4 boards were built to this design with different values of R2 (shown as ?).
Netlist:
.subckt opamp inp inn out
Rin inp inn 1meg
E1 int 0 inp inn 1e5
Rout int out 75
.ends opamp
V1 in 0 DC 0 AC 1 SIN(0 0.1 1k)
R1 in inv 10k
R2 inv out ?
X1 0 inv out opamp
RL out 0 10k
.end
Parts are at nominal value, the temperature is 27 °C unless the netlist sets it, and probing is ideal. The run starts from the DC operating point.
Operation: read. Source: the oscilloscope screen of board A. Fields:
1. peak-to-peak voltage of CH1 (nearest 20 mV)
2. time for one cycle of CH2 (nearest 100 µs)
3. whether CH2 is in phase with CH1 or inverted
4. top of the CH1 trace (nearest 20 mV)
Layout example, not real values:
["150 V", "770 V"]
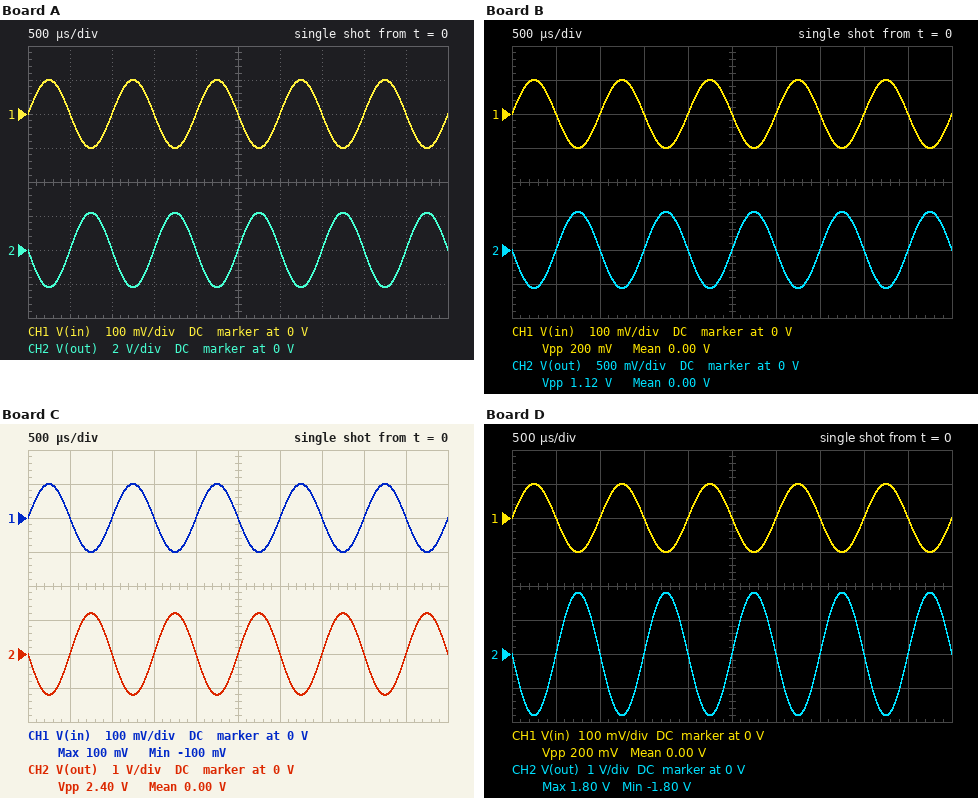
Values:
["200 mV", "1.0 ms", "inverted", "100 mV"]
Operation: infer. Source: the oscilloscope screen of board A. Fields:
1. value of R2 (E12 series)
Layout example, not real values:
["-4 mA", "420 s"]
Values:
["220 kΩ"]
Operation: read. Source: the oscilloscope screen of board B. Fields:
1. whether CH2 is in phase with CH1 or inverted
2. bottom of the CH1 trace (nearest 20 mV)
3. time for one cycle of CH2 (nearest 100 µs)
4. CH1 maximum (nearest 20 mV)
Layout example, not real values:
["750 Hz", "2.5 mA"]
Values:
["inverted", "-100 mV", "1.0 ms", "100 mV"]
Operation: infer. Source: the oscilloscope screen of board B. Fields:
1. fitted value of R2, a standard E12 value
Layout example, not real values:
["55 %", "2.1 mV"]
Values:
["56 kΩ"]
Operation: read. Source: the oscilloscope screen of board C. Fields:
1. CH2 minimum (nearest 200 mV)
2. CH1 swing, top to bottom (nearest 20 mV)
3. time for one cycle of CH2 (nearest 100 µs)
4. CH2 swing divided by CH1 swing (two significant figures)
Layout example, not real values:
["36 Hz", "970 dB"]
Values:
["-1.2 V", "200 mV", "1.0 ms", "12"]
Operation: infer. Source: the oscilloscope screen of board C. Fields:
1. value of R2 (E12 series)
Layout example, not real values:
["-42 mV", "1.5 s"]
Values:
["120 kΩ"]
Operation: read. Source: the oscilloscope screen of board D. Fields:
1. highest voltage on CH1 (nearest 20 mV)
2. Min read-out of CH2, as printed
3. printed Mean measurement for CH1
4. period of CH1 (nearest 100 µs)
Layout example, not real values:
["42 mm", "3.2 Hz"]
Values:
["100 mV", "-1.80 V", "0.00 V", "1.0 ms"]
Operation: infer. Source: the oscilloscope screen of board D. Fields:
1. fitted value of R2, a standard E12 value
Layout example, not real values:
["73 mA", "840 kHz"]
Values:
["180 kΩ"]
